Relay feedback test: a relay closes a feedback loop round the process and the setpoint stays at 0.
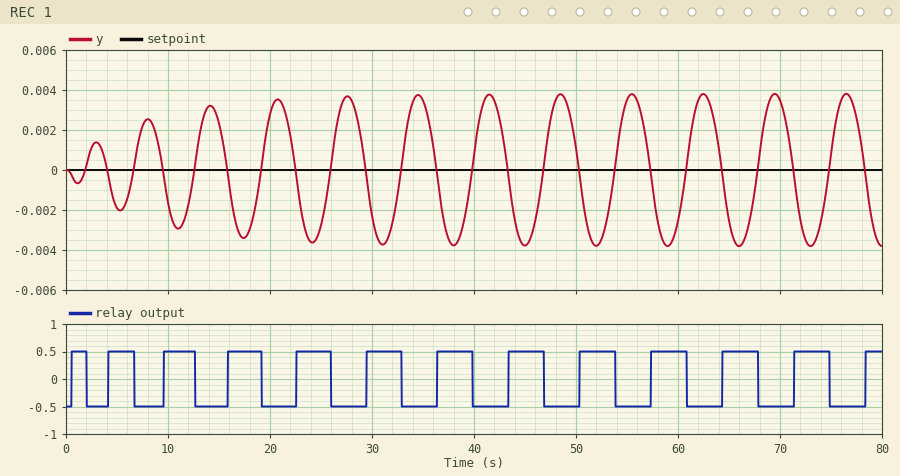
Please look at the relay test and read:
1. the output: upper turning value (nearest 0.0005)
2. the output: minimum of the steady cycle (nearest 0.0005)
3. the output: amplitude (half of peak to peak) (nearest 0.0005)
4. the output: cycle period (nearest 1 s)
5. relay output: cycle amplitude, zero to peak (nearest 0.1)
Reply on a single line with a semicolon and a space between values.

0.0040; -0.0040; 0.0040; 7 s; 0.5
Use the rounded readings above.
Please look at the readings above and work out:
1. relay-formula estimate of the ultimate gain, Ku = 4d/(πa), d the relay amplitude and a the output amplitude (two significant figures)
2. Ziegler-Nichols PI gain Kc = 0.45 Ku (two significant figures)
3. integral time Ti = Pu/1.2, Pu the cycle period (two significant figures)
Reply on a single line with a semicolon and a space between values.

160; 72; 5.8 s
